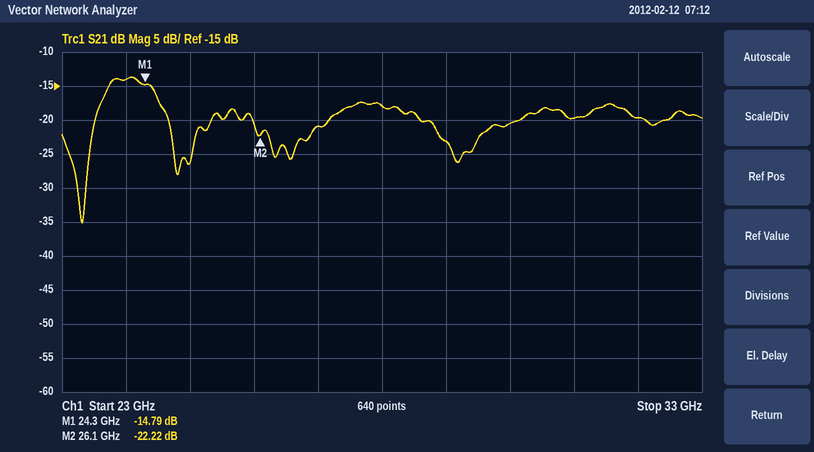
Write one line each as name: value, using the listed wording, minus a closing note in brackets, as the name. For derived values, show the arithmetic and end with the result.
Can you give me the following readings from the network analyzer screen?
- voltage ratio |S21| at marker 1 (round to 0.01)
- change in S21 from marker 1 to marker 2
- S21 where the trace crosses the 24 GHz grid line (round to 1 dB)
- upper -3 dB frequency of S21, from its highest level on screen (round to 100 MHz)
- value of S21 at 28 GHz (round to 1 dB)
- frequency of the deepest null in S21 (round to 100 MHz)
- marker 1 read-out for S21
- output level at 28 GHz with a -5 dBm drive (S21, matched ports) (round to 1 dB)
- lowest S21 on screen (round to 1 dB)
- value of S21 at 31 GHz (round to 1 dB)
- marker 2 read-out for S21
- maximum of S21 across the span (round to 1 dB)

voltage ratio |S21| at marker 1: 10^(-14.79/20) ≈ 0.18
change in S21 from marker 1 to marker 2: -22.22 − (-14.79) = -7.43 dB
S21 where the trace crosses the 24 GHz grid line: -14 dB
upper -3 dB frequency of S21, from its highest level on screen: 24.5 GHz
value of S21 at 28 GHz: -18 dB
frequency of the deepest null in S21: 23.3 GHz
marker 1 read-out for S21: -14.79 dB
output level at 28 GHz with a -5 dBm drive (S21, matched ports): -5 dBm + (-18 dB) = -23 dBm
lowest S21 on screen: -35 dB
value of S21 at 31 GHz: -20 dB
marker 2 read-out for S21: -22.22 dB
maximum of S21 across the span: -14 dB
